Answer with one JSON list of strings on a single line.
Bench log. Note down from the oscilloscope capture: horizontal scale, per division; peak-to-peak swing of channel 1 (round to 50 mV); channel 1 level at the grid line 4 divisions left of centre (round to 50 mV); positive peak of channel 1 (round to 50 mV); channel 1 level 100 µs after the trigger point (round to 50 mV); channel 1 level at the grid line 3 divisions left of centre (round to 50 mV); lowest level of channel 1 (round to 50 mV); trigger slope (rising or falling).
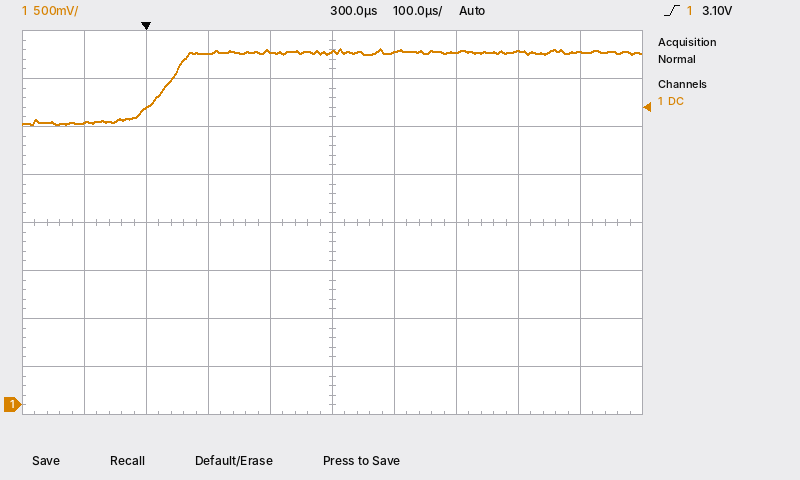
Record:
["100 µs", "800 mV", "2.95 V", "3.70 V", "3.65 V", "3.10 V", "2.90 V", "rising"]
